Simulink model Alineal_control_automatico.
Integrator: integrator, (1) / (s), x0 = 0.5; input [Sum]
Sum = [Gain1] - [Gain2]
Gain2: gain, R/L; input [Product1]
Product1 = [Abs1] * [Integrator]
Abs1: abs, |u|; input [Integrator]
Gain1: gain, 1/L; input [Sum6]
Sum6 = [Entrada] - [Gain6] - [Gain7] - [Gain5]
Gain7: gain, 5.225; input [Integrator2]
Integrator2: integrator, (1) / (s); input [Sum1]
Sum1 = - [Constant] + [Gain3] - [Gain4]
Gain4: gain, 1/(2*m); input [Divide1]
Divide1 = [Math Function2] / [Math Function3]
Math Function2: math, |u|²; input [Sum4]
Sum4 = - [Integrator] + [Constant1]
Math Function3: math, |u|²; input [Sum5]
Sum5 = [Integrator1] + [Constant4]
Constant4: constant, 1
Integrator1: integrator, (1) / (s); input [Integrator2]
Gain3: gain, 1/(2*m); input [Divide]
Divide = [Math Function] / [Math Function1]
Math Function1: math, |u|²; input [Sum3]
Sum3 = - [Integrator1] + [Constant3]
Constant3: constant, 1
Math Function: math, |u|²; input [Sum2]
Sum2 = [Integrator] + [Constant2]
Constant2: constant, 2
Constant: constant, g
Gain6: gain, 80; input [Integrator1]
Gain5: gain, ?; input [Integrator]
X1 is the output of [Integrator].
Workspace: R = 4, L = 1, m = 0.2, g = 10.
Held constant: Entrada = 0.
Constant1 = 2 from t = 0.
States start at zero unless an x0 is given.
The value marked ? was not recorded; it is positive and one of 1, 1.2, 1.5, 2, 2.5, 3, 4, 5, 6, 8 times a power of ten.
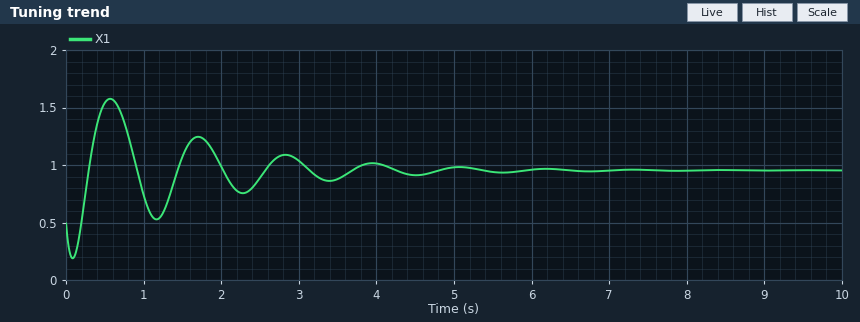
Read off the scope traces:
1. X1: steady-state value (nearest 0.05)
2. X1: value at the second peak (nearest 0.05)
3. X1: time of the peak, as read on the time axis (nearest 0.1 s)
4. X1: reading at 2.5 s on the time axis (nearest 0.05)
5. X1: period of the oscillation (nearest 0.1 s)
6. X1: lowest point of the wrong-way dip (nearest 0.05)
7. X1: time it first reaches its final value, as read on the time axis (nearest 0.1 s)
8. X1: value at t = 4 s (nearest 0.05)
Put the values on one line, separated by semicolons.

0.95; 1.25; 0.6 s; 0.90; 1.1 s; 0.20; 0.3 s; 1.00
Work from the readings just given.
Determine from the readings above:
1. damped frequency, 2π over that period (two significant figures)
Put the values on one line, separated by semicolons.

5.7 rad/s
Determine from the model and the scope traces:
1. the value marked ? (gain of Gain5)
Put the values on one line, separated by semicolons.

15
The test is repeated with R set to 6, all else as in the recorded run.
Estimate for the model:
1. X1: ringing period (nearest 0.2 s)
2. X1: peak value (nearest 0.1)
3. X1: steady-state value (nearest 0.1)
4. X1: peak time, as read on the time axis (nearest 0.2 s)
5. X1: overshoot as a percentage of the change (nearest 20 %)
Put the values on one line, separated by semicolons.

1.4 s; 1.7; 1.1; 0.6 s; 100 %
